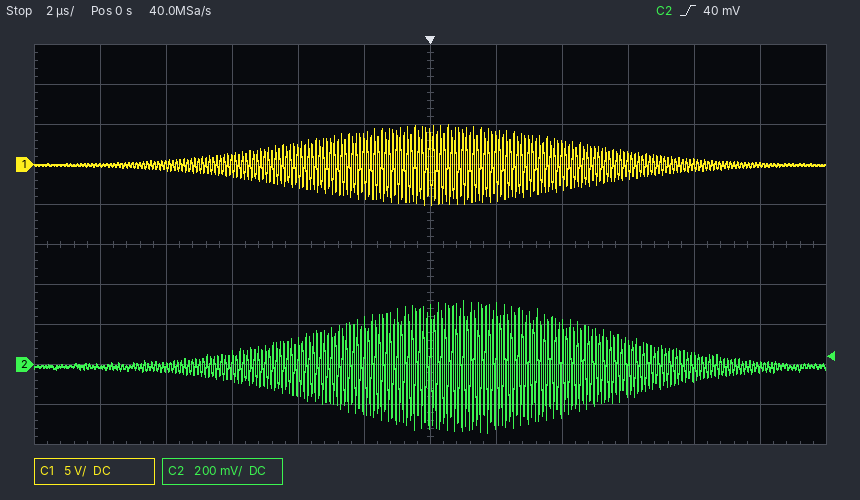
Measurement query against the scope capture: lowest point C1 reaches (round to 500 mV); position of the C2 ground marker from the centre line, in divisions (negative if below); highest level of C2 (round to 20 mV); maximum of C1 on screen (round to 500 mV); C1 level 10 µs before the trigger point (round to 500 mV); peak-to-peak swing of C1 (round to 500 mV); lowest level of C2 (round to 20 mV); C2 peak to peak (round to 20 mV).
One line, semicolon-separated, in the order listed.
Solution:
-5.0 V; -3.0 div; 320 mV; 5.0 V; 0.0 V; 10.0 V; -340 mV; 660 mV
